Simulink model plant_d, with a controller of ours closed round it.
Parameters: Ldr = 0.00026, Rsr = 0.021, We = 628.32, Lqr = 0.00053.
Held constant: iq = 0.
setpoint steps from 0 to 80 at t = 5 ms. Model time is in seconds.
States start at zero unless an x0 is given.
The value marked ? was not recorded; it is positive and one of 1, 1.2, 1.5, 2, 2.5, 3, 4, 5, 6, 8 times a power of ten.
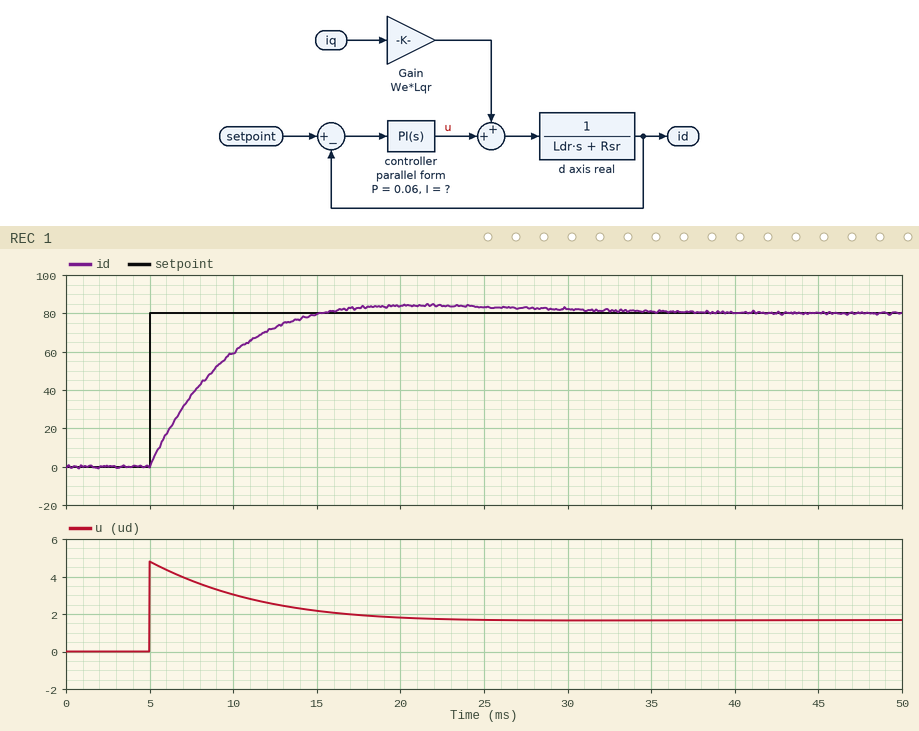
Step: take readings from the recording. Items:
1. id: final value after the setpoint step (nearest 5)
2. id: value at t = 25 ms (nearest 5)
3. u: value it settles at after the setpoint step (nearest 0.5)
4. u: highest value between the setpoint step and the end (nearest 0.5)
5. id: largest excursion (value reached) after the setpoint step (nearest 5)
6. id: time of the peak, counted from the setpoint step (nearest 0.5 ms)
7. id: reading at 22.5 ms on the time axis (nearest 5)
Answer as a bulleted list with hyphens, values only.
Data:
- 80
- 85
- 1.5
- 5.0
- 85
- 16.0 ms
- 85
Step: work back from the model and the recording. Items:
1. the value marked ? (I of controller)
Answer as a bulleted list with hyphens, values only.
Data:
- 8
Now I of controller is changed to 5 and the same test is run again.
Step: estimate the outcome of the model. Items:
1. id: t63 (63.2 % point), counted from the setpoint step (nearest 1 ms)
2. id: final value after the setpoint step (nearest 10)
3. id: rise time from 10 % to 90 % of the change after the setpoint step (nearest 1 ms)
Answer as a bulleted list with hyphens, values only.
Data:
- 4 ms
- 80
- 9 ms
